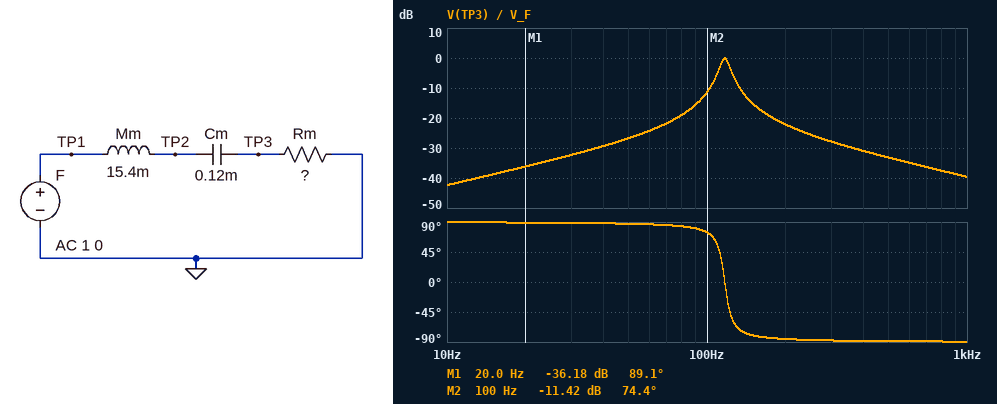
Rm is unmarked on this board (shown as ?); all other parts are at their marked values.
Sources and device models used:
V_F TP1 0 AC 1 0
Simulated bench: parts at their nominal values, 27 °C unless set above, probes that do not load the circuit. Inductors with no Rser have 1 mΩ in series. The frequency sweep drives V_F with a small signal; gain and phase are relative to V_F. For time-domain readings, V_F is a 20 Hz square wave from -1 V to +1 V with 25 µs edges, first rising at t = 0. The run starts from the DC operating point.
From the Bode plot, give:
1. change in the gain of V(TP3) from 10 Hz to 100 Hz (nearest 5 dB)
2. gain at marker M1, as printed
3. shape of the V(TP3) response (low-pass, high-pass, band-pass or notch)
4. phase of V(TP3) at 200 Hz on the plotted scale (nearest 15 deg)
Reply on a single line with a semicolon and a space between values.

30 dB; -36.18 dB; band-pass; -90 deg
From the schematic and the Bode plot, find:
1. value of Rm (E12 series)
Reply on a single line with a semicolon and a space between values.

1 Ω
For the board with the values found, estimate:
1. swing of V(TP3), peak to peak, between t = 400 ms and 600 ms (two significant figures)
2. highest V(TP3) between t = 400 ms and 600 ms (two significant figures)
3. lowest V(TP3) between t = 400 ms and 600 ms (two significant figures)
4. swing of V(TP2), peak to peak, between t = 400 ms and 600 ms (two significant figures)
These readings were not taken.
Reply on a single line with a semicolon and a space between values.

240 mV; 120 mV; -120 mV; 4.5 V
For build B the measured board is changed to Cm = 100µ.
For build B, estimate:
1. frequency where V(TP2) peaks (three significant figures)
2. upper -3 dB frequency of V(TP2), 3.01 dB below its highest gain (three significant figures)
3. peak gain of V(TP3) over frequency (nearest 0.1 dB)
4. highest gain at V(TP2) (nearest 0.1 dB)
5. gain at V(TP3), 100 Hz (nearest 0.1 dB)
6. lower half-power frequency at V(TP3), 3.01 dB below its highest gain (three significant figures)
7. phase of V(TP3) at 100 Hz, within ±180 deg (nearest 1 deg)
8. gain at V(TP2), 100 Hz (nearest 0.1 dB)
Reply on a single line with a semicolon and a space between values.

128 Hz; 133 Hz; 0 dB; 21.9 dB; -16.0 dB; 123 Hz; 81 deg; 8.0 dB
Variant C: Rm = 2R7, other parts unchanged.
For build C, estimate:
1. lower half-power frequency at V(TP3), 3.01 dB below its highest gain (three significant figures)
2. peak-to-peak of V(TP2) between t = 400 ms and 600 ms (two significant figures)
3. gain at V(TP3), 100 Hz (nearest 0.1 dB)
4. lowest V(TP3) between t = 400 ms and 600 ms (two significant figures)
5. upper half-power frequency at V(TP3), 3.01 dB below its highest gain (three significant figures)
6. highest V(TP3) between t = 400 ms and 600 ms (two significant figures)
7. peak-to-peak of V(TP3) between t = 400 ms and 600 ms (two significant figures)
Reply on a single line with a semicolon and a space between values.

104 Hz; 4.6 V; -4.4 dB; -370 mV; 132 Hz; 370 mV; 740 mV
